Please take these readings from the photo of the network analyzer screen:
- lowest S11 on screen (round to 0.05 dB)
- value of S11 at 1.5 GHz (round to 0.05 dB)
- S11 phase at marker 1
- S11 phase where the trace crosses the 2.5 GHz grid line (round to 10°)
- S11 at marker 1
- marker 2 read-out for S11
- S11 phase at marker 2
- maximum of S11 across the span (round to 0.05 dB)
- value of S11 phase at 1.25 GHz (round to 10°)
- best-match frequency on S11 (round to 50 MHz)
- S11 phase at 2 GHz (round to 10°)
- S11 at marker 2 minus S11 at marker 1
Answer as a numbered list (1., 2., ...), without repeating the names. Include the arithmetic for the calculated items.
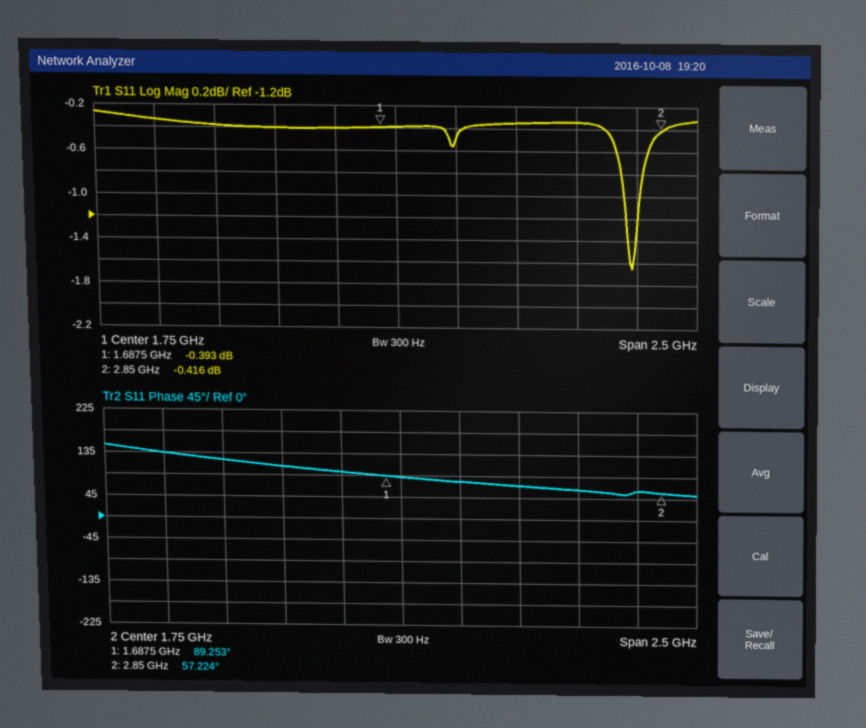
1. -1.65 dB
2. -0.40 dB
3. 89.253°
4. 60°
5. -0.393 dB
6. -0.416 dB
7. 57.224°
8. -0.25 dB
9. 110°
10. 2.75 GHz
11. 80°
12. -0.416 − (-0.393) = -0.023 dB
